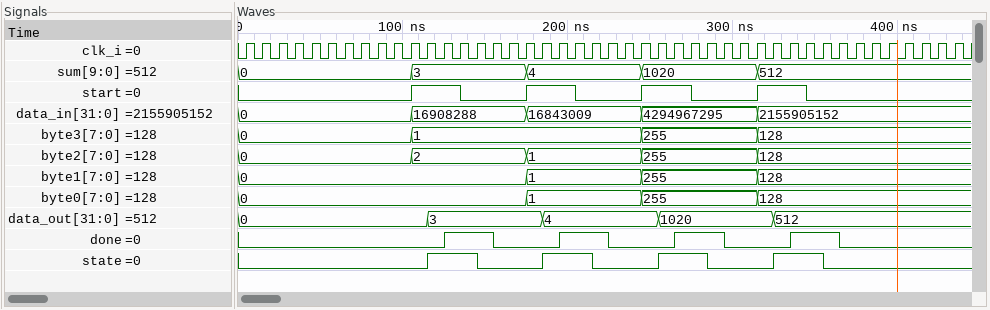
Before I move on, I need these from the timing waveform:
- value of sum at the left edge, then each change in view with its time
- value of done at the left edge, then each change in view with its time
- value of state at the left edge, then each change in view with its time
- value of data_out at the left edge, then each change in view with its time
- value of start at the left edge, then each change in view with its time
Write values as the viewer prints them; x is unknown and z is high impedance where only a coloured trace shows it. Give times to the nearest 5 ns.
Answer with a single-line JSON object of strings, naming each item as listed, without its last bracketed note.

{"value of sum at the left edge, then each change in view with its time": "0, 3 at 105 ns, 4 at 175 ns, 1020 at 245 ns, 512 at 315 ns", "value of done at the left edge, then each change in view with its time": "0, 1 at 125 ns, 0 at 155 ns, 1 at 195 ns, 0 at 225 ns, 1 at 265 ns, 0 at 295 ns, 1 at 335 ns, 0 at 365 ns", "value of state at the left edge, then each change in view with its time": "0, 1 at 115 ns, 0 at 145 ns, 1 at 185 ns, 0 at 215 ns, 1 at 255 ns, 0 at 285 ns, 1 at 325 ns, 0 at 355 ns", "value of data_out at the left edge, then each change in view with its time": "0, 3 at 115 ns, 4 at 185 ns, 1020 at 255 ns, 512 at 325 ns", "value of start at the left edge, then each change in view with its time": "0, 1 at 105 ns, 0 at 135 ns, 1 at 175 ns, 0 at 205 ns, 1 at 245 ns, 0 at 275 ns, 1 at 315 ns, 0 at 345 ns"}
